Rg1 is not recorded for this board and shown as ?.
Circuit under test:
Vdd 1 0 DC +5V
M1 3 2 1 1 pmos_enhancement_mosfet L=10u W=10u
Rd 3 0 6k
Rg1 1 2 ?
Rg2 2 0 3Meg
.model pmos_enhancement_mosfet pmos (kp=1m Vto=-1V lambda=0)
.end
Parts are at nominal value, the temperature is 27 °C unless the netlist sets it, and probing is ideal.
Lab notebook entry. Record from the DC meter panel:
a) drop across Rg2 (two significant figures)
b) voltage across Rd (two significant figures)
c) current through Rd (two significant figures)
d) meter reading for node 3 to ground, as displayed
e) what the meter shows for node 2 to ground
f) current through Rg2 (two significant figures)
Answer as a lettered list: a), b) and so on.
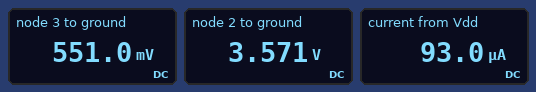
a) 3.6 V
b) 550 mV
c) 92 µA
d) 551.0 mV
e) 3.571 V
f) 1.2 µA
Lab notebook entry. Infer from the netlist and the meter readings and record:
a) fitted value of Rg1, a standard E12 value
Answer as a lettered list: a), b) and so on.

a) 1.2 MΩ
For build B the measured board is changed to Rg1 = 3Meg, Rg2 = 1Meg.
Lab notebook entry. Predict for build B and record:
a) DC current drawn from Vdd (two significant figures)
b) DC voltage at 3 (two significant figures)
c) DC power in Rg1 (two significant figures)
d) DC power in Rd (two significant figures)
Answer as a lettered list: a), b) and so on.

a) 780 µA
b) 4.7 V
c) 4.7 µW
d) 3.7 mW
